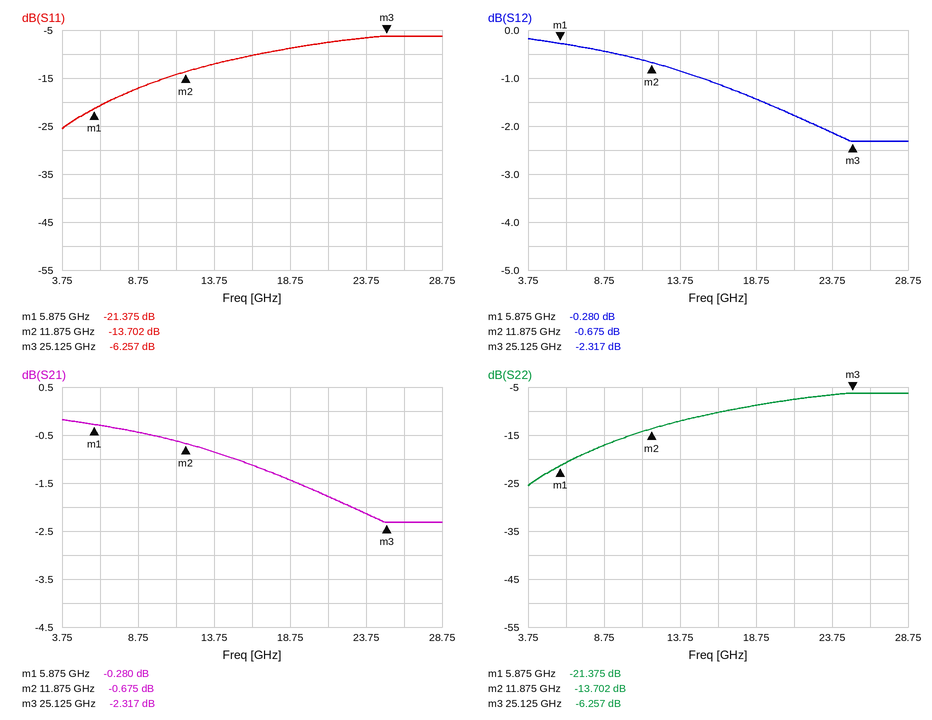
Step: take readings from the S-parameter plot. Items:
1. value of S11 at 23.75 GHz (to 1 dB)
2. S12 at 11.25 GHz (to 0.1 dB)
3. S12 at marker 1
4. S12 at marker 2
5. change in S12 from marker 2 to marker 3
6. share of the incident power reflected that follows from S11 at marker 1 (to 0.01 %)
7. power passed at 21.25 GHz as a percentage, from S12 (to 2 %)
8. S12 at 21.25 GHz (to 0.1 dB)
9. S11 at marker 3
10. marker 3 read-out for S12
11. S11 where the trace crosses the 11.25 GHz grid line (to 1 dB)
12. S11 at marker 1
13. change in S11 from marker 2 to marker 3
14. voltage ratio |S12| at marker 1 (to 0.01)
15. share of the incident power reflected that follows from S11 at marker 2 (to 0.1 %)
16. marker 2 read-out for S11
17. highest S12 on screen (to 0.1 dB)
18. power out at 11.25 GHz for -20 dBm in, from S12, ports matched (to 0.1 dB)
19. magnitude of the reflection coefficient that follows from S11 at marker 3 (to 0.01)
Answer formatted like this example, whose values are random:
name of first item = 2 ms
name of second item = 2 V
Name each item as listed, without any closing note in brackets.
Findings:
value of S11 at 23.75 GHz = -7 dB
S12 at 11.25 GHz = -0.6 dB
S12 at marker 1 = -0.280 dB
S12 at marker 2 = -0.675 dB
change in S12 from marker 2 to marker 3 = -1.642 dB
share of the incident power reflected that follows from S11 at marker 1 = 0.73 %
power passed at 21.25 GHz as a percentage, from S12 = 66 %
S12 at 21.25 GHz = -1.8 dB
S11 at marker 3 = -6.257 dB
marker 3 read-out for S12 = -2.317 dB
S11 where the trace crosses the 11.25 GHz grid line = -14 dB
S11 at marker 1 = -21.375 dB
change in S11 from marker 2 to marker 3 = 7.445 dB
voltage ratio |S12| at marker 1 = 0.97
share of the incident power reflected that follows from S11 at marker 2 = 4.3 %
marker 2 read-out for S11 = -13.702 dB
highest S12 on screen = -0.2 dB
power out at 11.25 GHz for -20 dBm in, from S12, ports matched = -20.6 dBm
magnitude of the reflection coefficient that follows from S11 at marker 3 = 0.49
